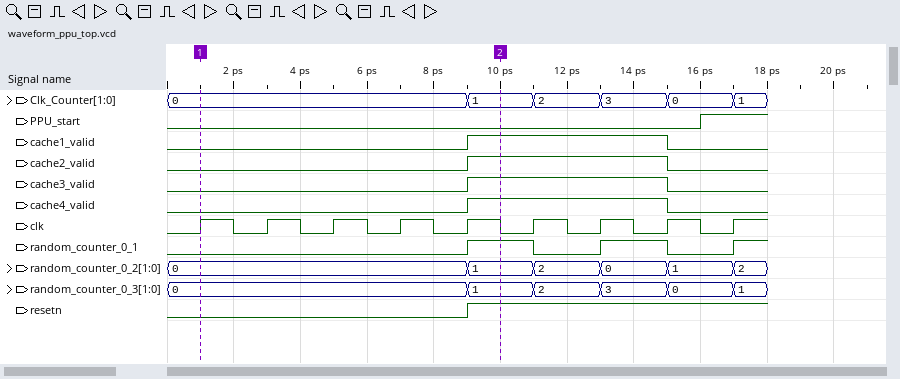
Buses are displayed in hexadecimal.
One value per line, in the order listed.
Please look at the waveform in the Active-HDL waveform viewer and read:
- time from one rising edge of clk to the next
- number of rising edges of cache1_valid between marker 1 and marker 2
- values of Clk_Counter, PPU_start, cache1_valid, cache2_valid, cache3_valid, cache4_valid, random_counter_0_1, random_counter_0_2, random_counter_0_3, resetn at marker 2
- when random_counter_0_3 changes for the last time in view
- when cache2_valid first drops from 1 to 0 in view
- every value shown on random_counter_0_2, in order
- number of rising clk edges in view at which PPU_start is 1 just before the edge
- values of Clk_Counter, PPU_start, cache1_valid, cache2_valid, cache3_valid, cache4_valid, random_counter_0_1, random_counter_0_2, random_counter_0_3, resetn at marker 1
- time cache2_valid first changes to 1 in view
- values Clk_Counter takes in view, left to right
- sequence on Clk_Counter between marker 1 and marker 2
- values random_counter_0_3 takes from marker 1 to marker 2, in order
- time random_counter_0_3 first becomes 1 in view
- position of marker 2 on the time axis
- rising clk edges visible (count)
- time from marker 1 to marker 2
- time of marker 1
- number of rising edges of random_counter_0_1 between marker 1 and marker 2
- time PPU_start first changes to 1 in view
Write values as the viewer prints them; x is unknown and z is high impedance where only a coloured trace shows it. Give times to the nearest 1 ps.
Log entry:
2 ps
1
Clk_Counter=1, PPU_start=0, cache1_valid=1, cache2_valid=1, cache3_valid=1, cache4_valid=1, random_counter_0_1=1, random_counter_0_2=1, random_counter_0_3=1, resetn=1
17 ps
15 ps
0, 1, 2, 0, 1, 2
1
Clk_Counter=0, PPU_start=0, cache1_valid=0, cache2_valid=0, cache3_valid=0, cache4_valid=0, random_counter_0_1=0, random_counter_0_2=0, random_counter_0_3=0, resetn=0
9 ps
0, 1, 2, 3, 0, 1
0, 1
0, 1
9 ps
10 ps
9
9 ps
1 ps
1
16 ps
